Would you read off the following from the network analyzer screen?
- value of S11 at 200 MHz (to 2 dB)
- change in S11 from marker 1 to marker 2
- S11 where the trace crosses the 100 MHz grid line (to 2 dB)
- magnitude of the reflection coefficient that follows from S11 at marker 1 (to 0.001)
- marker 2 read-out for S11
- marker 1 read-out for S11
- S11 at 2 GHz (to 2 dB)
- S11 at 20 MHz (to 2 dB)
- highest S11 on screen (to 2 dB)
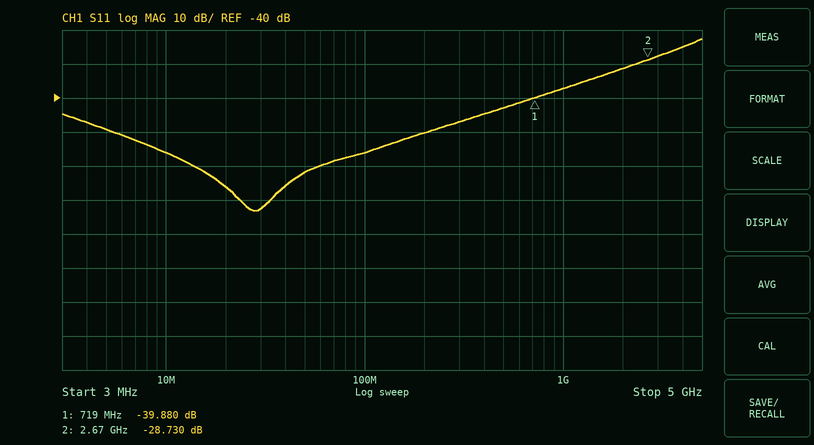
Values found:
-50 dB
11.150 dB
-56 dB
0.010
-28.730 dB
-39.880 dB
-32 dB
-66 dB
-22 dB
